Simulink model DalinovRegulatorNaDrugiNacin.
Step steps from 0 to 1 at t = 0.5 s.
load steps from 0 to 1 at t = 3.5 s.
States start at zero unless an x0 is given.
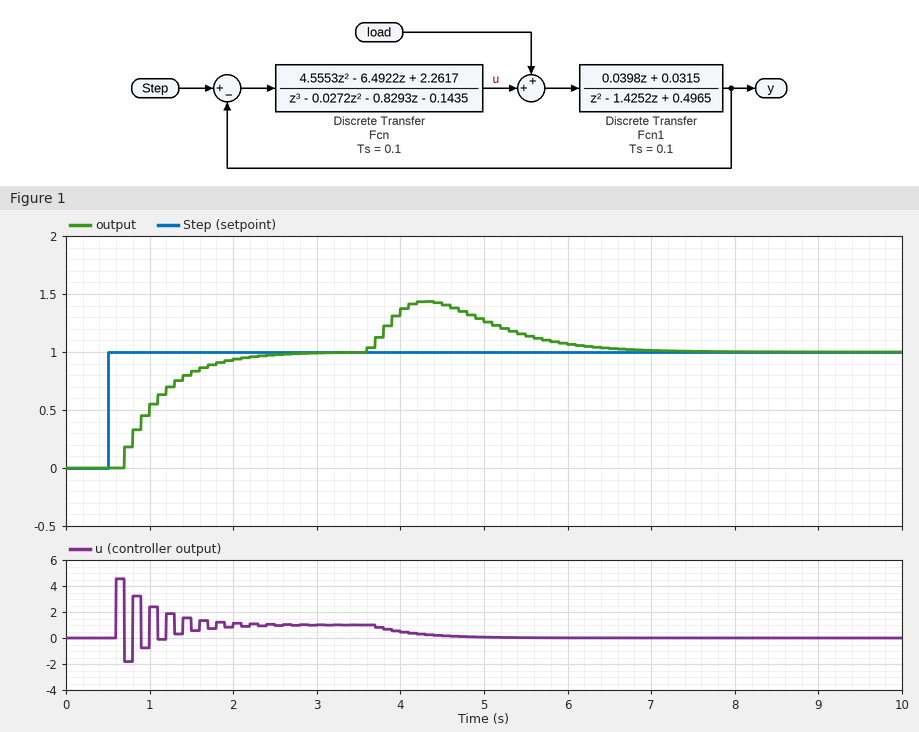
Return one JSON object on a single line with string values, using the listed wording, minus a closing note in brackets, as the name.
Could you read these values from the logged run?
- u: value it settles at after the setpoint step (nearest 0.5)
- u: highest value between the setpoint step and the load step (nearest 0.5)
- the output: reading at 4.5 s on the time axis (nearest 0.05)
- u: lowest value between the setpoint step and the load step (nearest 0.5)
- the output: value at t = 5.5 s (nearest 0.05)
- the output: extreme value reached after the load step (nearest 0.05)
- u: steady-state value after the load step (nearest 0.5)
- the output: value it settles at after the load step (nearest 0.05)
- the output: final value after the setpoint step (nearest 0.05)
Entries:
{"u: value it settles at after the setpoint step": "1.0", "u: highest value between the setpoint step and the load step": "4.5", "the output: reading at 4.5 s on the time axis": "1.40", "u: lowest value between the setpoint step and the load step": "-2.0", "the output: value at t = 5.5 s": "1.15", "the output: extreme value reached after the load step": "1.45", "u: steady-state value after the load step": "0.0", "the output: value it settles at after the load step": "1.00", "the output: final value after the setpoint step": "1.00"}
